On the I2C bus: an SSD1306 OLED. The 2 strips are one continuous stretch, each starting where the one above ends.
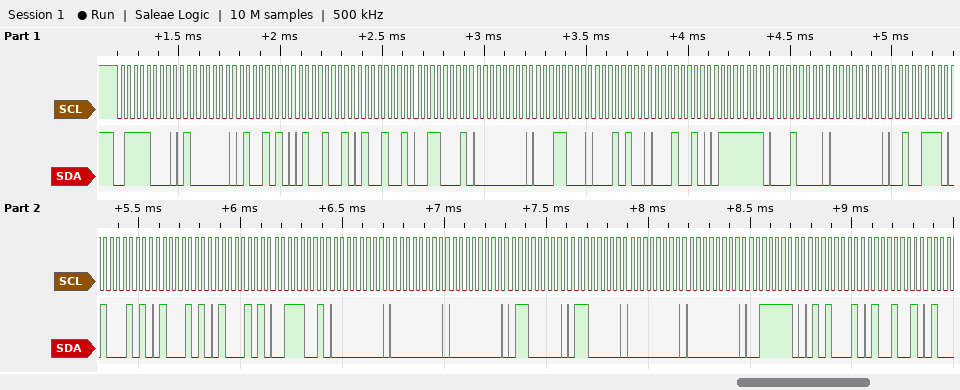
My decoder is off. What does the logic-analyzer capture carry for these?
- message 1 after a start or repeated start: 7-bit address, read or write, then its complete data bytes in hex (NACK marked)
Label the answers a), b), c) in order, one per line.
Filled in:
a) 0x3C write: 40 4A 49 49 31 00 18 14 12 7F 10 00 27 45 45 45 39 00 00 00 60 60 00 00 3E 51 49
